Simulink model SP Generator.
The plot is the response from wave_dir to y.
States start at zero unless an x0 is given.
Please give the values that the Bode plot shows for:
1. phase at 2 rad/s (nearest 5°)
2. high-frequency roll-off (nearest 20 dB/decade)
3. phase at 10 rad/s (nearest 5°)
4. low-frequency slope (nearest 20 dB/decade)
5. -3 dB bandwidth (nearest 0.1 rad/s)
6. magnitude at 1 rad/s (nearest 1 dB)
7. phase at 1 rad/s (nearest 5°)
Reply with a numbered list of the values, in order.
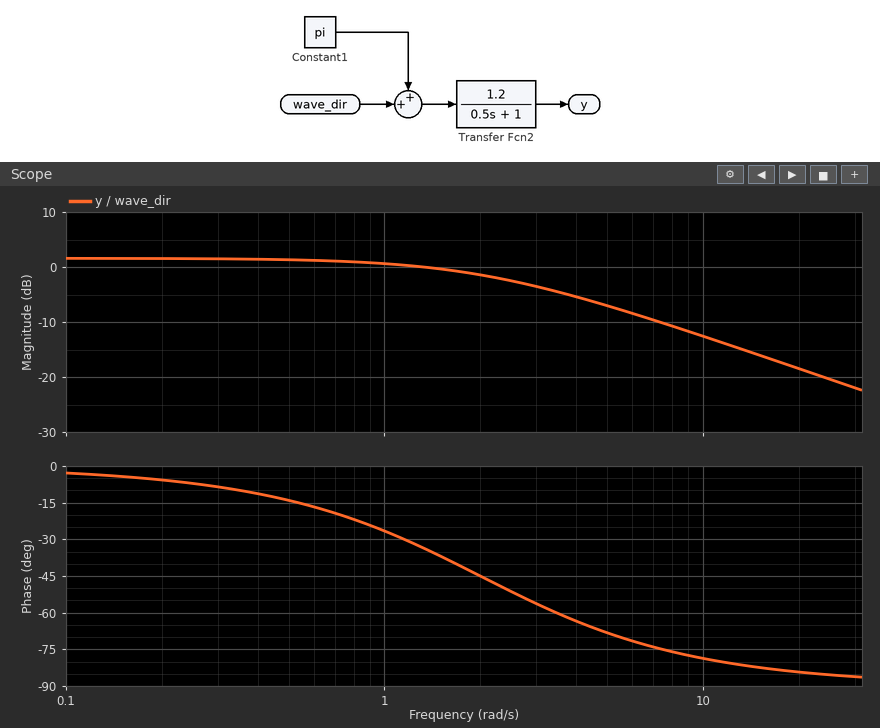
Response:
1. -45°
2. -20 dB/decade
3. -80°
4. 0 dB/decade
5. 2.0 rad/s
6. 1 dB
7. -25°
